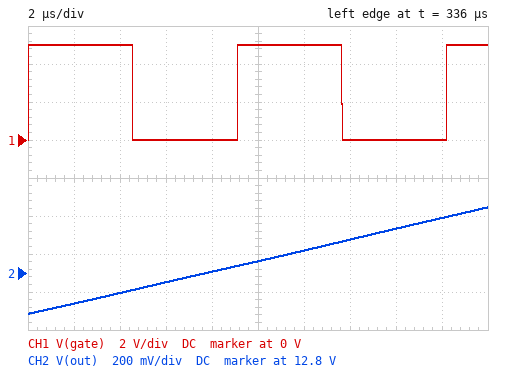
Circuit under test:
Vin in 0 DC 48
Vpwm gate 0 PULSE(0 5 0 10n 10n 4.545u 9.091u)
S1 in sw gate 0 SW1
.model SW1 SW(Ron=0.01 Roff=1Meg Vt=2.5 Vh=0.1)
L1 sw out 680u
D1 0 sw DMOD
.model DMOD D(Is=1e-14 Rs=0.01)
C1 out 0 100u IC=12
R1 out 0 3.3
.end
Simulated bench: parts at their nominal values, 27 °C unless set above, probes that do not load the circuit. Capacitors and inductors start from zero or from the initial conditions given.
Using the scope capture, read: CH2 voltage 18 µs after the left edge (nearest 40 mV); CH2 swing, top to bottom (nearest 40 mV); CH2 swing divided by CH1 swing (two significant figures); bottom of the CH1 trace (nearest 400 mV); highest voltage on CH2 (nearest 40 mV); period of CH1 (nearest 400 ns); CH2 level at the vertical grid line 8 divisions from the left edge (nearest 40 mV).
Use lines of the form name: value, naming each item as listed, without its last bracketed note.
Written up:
CH2 voltage 18 µs after the left edge: 13.08 V
CH2 swing, top to bottom: 560 mV
CH2 swing divided by CH1 swing: 0.11
bottom of the CH1 trace: 0 V
highest voltage on CH2: 13.16 V
period of CH1: 9.2 µs
CH2 level at the vertical grid line 8 divisions from the left edge: 13.04 V
